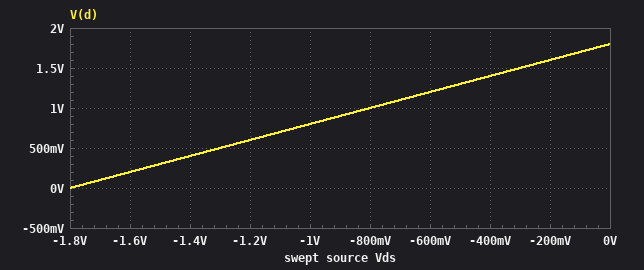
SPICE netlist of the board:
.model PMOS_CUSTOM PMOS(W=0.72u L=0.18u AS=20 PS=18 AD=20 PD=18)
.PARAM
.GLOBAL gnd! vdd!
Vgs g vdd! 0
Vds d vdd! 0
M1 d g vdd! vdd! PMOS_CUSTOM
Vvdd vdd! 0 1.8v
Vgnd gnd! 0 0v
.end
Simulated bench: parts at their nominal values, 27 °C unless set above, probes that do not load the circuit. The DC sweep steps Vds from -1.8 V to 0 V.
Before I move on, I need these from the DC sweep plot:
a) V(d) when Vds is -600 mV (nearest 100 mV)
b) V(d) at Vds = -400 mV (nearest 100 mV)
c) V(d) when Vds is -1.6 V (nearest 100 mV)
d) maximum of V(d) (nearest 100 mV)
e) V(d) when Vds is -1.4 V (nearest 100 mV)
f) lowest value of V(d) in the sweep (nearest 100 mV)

1.2 V
1.4 V
200 mV
1.8 V
400 mV
0 V
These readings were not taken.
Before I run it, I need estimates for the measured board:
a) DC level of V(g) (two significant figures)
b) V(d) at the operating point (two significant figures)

1.8 V
1.8 V
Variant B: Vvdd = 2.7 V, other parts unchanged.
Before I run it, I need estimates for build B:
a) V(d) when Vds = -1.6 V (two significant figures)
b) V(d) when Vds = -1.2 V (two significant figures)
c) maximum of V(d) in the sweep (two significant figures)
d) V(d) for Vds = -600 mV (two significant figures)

1.1 V
1.5 V
2.7 V
2.1 V
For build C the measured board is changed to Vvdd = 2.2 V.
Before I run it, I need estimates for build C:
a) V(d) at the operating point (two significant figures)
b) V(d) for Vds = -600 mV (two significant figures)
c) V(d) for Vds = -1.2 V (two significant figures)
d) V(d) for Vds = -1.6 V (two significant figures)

2.2 V
1.6 V
1.0 V
600 mV
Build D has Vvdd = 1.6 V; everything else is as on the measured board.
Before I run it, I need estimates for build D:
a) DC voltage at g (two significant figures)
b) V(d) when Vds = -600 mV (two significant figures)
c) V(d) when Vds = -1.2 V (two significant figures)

1.6 V
1.0 V
400 mV
